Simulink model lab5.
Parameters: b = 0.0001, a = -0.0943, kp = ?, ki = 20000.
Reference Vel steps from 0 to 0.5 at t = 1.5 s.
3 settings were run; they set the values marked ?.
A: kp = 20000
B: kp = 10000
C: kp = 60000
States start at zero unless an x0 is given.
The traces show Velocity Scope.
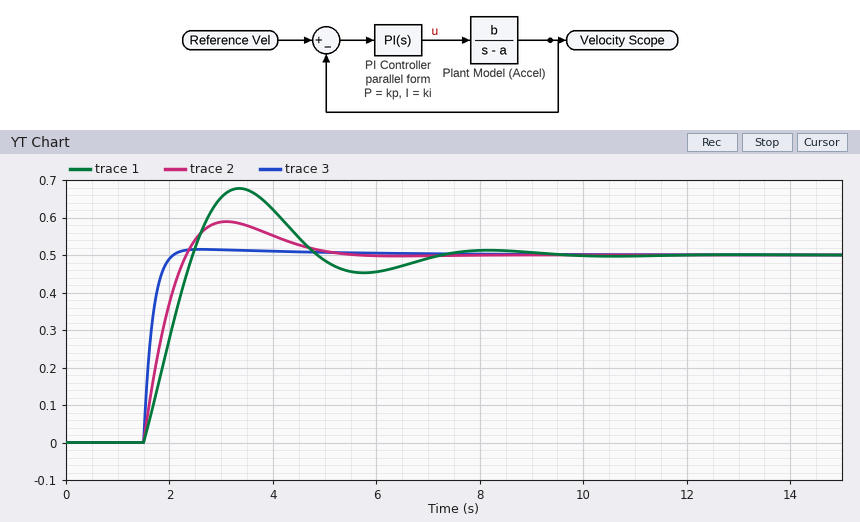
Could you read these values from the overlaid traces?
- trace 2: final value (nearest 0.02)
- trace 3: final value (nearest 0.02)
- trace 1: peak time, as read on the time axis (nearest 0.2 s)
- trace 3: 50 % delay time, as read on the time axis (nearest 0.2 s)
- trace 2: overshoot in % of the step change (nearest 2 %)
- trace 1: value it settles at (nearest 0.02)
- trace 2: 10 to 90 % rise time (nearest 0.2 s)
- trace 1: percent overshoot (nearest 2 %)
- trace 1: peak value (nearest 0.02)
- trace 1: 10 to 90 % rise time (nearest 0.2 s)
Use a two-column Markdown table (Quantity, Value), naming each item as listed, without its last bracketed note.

| Quantity | Value |
|---|---|
| trace 2: final value | 0.50 |
| trace 3: final value | 0.50 |
| trace 1: peak time, as read on the time axis | 3.4 s |
| trace 3: 50 % delay time, as read on the time axis | 1.6 s |
| trace 2: overshoot in % of the step change | 18 % |
| trace 1: value it settles at | 0.50 |
| trace 2: 10 to 90 % rise time | 0.6 s |
| trace 1: percent overshoot | 36 % |
| trace 1: peak value | 0.68 |
| trace 1: 10 to 90 % rise time | 0.8 s |
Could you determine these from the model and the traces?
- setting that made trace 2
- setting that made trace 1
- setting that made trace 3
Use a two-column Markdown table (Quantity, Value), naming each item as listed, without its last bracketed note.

| Quantity | Value |
|---|---|
| setting that made trace 2 | A |
| setting that made trace 1 | B |
| setting that made trace 3 | C |
